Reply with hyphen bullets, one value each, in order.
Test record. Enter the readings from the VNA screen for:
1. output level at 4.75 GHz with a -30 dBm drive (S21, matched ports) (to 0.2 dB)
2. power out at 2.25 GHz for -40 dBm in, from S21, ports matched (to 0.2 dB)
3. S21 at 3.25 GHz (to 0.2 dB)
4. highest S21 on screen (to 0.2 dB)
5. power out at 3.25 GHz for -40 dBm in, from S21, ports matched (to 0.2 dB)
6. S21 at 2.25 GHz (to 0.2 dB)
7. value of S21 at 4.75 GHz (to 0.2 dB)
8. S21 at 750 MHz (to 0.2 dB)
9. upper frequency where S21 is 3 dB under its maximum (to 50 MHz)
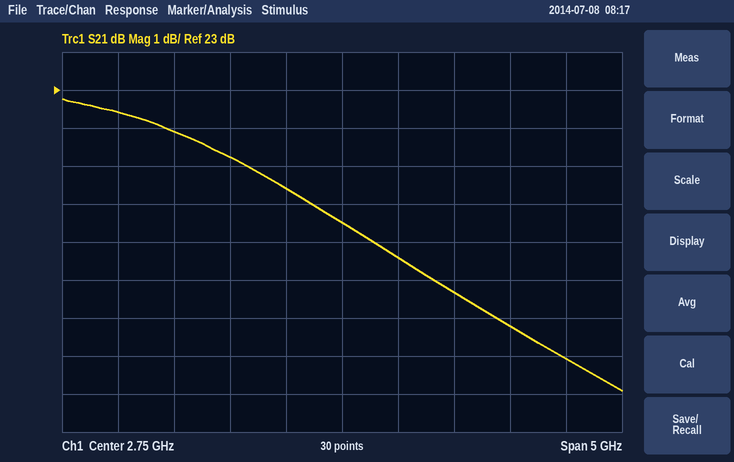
- -14.0 dBm
- -19.6 dBm
- 18.6 dB
- 22.8 dB
- -21.4 dBm
- 20.4 dB
- 16.0 dB
- 22.4 dB
- 2.60 GHz
